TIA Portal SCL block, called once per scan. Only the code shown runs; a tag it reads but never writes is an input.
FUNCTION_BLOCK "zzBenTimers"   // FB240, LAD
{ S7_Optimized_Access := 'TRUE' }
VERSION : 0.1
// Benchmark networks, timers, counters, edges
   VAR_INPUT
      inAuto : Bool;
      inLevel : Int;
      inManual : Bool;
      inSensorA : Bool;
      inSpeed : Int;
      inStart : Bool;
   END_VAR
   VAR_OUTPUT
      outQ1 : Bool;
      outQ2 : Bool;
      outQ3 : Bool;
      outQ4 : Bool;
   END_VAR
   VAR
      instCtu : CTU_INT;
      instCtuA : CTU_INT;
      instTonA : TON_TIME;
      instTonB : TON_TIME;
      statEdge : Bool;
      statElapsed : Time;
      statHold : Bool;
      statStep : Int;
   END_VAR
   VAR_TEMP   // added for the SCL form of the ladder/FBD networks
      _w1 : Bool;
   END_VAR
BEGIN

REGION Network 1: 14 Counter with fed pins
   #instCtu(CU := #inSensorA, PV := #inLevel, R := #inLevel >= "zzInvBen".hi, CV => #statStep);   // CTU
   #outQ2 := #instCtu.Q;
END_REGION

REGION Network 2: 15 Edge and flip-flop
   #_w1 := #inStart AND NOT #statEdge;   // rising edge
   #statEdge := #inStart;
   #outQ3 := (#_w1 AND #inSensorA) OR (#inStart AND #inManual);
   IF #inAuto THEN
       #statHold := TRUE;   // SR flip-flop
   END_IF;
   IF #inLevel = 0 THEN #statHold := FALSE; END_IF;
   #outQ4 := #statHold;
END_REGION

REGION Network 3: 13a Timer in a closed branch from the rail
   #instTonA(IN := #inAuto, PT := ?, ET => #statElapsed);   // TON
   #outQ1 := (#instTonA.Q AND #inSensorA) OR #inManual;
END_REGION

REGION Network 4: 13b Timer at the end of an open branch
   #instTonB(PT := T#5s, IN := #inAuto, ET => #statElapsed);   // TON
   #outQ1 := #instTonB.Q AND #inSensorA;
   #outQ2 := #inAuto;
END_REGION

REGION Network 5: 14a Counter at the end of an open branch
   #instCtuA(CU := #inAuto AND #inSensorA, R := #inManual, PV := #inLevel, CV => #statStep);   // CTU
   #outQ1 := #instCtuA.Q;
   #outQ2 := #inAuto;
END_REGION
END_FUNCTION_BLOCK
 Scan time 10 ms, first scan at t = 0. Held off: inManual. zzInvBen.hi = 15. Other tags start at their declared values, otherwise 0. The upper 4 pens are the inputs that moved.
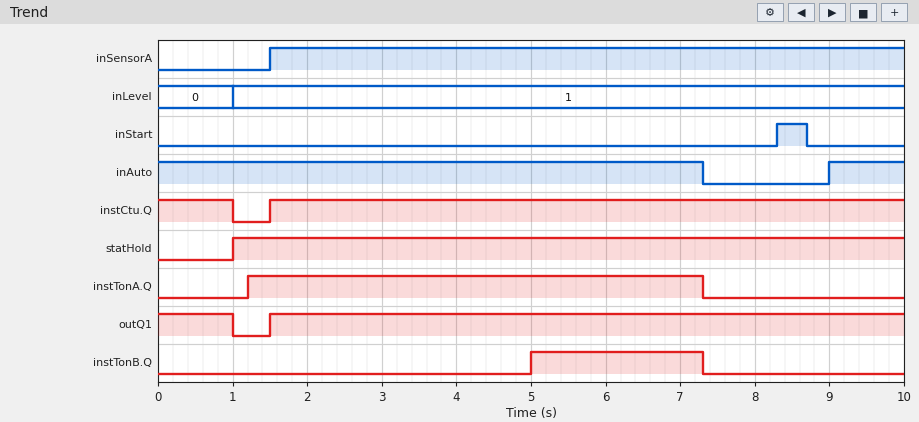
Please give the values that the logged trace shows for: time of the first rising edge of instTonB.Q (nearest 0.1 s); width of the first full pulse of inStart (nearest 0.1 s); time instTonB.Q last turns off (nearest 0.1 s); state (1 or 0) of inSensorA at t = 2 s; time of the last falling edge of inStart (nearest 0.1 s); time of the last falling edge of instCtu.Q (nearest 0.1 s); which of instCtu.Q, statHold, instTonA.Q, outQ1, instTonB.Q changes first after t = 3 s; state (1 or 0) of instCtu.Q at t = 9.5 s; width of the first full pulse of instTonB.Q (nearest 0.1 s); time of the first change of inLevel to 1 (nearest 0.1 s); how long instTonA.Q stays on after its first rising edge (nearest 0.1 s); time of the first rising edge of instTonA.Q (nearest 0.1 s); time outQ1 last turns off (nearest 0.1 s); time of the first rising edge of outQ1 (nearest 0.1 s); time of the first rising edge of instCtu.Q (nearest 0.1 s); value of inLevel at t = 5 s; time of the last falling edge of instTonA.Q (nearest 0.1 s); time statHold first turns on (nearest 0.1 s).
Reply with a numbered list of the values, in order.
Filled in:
1. 5.0 s
2. 0.4 s
3. 7.3 s
4. 1
5. 8.7 s
6. 1.0 s
7. instTonB.Q
8. 1
9. 2.3 s
10. 1.0 s
11. 6.1 s
12. 1.2 s
13. 1.0 s
14. 1.5 s
15. 1.5 s
16. 1
17. 7.3 s
18. 1.0 s
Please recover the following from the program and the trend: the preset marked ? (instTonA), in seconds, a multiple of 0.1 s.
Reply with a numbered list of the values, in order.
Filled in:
1. 1.2 s
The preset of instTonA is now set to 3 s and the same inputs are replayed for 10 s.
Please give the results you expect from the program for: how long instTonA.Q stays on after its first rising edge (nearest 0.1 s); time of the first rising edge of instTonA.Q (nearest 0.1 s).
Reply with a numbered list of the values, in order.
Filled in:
1. 4.3 s
2. 3.0 s
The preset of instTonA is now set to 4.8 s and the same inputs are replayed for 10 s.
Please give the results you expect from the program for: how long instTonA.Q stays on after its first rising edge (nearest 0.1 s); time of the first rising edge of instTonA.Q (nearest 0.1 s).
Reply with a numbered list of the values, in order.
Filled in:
1. 2.5 s
2. 4.8 s
